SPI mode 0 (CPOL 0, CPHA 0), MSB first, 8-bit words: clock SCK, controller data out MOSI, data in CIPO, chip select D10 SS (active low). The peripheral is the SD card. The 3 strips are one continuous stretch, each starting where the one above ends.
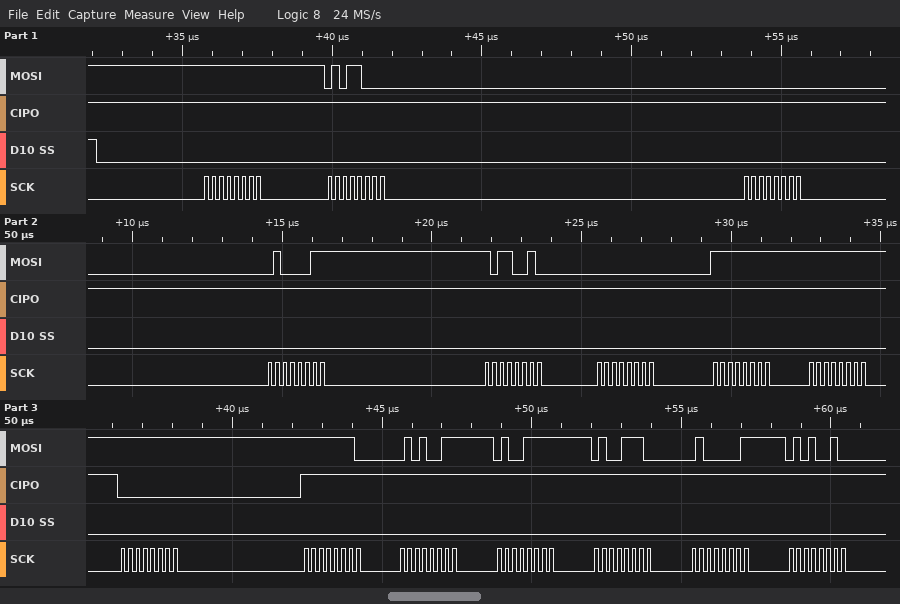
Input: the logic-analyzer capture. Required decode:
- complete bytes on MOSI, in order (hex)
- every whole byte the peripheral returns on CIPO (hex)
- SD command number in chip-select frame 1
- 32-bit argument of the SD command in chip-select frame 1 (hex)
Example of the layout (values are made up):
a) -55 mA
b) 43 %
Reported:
a) FF 58 00 43 B2 00 FF FF FF FE 53 4F 4E 41 52
b) FF FF FF FF FF FF FF FF 00 FF FF FF FF FF FF
c) CMD24
d) 0x0043B200
